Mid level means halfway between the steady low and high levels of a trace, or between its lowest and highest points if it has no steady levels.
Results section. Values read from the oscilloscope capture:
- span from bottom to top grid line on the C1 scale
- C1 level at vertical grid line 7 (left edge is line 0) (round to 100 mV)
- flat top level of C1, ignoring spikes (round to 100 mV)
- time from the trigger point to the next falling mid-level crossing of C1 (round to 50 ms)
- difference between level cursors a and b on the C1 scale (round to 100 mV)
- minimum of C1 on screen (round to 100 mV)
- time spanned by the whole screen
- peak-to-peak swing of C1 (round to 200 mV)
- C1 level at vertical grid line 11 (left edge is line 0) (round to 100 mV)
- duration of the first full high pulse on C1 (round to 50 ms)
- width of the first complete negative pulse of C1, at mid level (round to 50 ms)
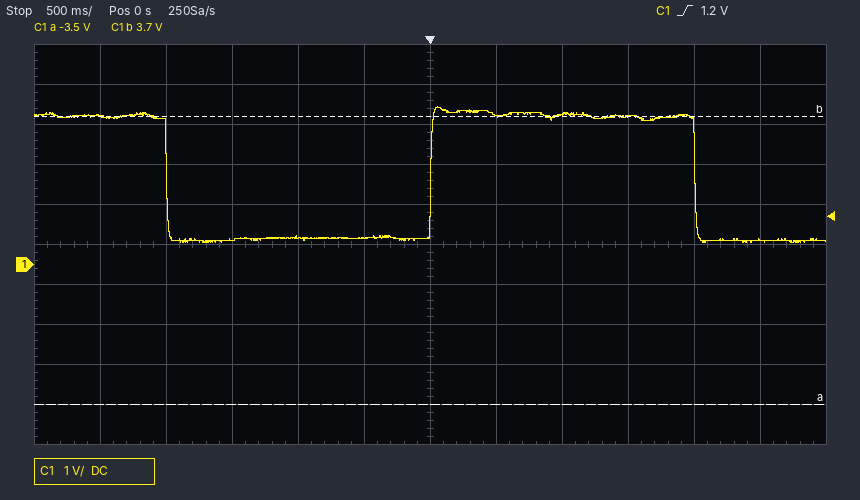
10 V
3.7 V
3.7 V
2.00 s
7.2 V
600 mV
6 s
3.4 V
600 mV
2.00 s
2.00 s
